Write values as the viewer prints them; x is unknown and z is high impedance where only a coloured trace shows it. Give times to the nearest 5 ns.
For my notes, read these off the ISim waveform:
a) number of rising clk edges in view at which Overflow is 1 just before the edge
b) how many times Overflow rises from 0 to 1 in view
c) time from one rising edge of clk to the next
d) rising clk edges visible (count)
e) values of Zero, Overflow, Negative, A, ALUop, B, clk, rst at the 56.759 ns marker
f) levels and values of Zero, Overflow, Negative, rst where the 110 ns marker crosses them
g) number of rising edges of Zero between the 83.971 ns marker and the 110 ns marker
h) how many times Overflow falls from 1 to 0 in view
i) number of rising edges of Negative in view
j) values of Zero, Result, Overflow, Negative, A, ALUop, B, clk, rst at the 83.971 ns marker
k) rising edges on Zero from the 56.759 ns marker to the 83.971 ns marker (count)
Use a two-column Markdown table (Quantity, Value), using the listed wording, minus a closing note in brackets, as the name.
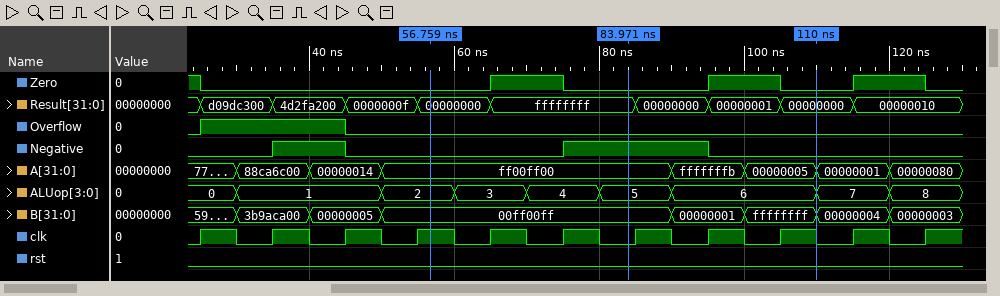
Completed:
| Quantity | Value |
|---|---|
| number of rising clk edges in view at which Overflow is 1 just before the edge | 2 |
| how many times Overflow rises from 0 to 1 in view | 1 |
| time from one rising edge of clk to the next | 10 ns |
| rising clk edges visible | 11 |
| values of Zero, Overflow, Negative, A, ALUop, B, clk, rst at the 56.759 ns marker | Zero=0, Overflow=0, Negative=0, A=ff00ff00, ALUop=2, B=00ff00ff, clk=1, rst=0 |
| levels and values of Zero, Overflow, Negative, rst where the 110 ns marker crosses them | Zero=0, Overflow=0, Negative=0, rst=0 |
| number of rising edges of Zero between the 83.971 ns marker and the 110 ns marker | 1 |
| how many times Overflow falls from 1 to 0 in view | 1 |
| number of rising edges of Negative in view | 2 |
| values of Zero, Result, Overflow, Negative, A, ALUop, B, clk, rst at the 83.971 ns marker | Zero=0, Result=ffffffff, Overflow=0, Negative=1, A=ff00ff00, ALUop=5, B=00ff00ff, clk=0, rst=0 |
| rising edges on Zero from the 56.759 ns marker to the 83.971 ns marker | 1 |
